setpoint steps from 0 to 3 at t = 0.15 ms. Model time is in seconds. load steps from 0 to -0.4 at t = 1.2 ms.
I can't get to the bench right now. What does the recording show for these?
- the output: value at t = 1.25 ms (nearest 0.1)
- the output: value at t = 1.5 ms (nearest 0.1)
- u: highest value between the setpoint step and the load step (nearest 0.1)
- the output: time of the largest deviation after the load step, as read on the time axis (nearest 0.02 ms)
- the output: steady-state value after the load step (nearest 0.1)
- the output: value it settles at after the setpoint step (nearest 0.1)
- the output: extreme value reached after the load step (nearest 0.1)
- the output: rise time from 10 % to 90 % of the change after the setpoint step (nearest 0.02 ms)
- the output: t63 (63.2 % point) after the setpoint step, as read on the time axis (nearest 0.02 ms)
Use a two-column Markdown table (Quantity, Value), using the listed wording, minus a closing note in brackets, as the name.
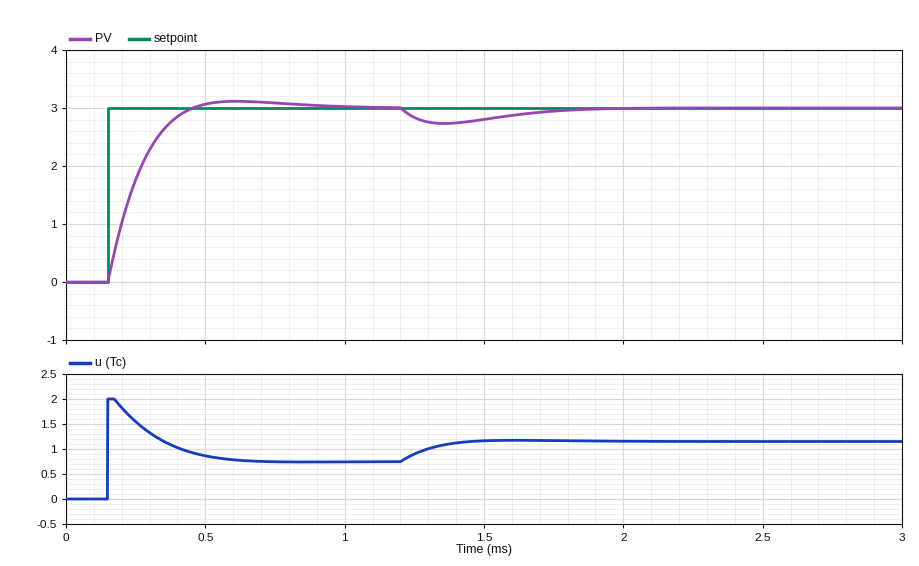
| Quantity | Value |
|---|---|
| the output: value at t = 1.25 ms | 2.8 |
| the output: value at t = 1.5 ms | 2.8 |
| u: highest value between the setpoint step and the load step | 2.0 |
| the output: time of the largest deviation after the load step, as read on the time axis | 1.36 ms |
| the output: steady-state value after the load step | 3.0 |
| the output: value it settles at after the setpoint step | 3.0 |
| the output: extreme value reached after the load step | 2.7 |
| the output: rise time from 10 % to 90 % of the change after the setpoint step | 0.20 ms |
| the output: t63 (63.2 % point) after the setpoint step, as read on the time axis | 0.26 ms |
